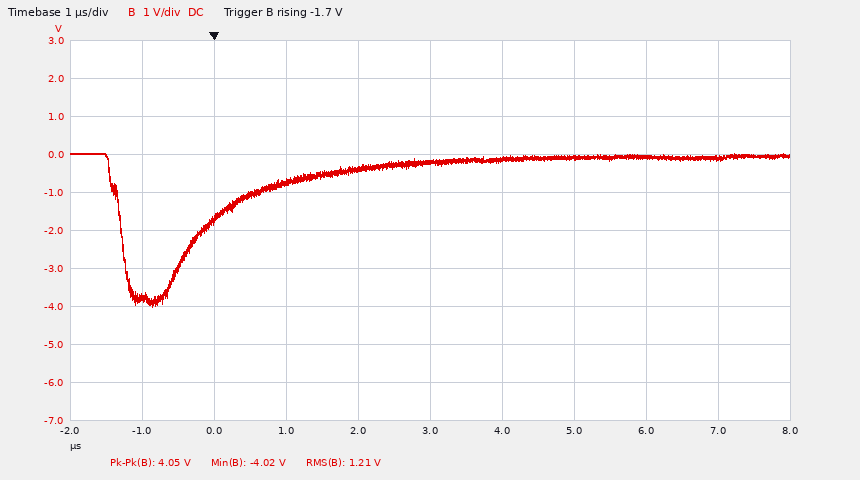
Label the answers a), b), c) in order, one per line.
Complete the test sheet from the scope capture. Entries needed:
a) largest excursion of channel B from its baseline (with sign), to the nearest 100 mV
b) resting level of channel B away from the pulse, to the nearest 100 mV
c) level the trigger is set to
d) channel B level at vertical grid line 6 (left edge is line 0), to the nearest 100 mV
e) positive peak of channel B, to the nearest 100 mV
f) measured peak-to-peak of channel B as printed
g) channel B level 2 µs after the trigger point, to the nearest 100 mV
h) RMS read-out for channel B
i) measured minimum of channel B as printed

a) -3.9 V
b) -100 mV
c) -1.7 V
d) -100 mV
e) 0.0 V
f) 4.05 V
g) -400 mV
h) 1.21 V
i) -4.02 V
